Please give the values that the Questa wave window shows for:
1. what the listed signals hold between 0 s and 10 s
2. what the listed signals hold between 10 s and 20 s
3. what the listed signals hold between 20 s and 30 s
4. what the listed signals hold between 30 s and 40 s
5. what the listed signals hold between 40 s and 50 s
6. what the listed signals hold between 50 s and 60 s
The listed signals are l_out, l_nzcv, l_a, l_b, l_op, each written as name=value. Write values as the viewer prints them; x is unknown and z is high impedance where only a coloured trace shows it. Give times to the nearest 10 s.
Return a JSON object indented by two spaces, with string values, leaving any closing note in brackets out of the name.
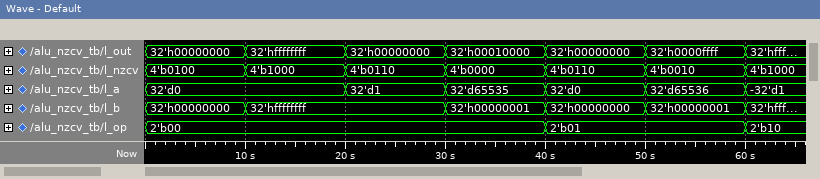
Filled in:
{
  "what the listed signals hold between 0 s and 10 s": "l_out=32'h00000000, l_nzcv=4'b0100, l_a=32'd0, l_b=32'h00000000, l_op=2'b00",
  "what the listed signals hold between 10 s and 20 s": "l_out=32'hffffffff, l_nzcv=4'b1000, l_a=32'd0, l_b=32'hffffffff, l_op=2'b00",
  "what the listed signals hold between 20 s and 30 s": "l_out=32'h00000000, l_nzcv=4'b0110, l_a=32'd1, l_b=32'hffffffff, l_op=2'b00",
  "what the listed signals hold between 30 s and 40 s": "l_out=32'h00010000, l_nzcv=4'b0000, l_a=32'd65535, l_b=32'h00000001, l_op=2'b00",
  "what the listed signals hold between 40 s and 50 s": "l_out=32'h00000000, l_nzcv=4'b0110, l_a=32'd0, l_b=32'h00000000, l_op=2'b01",
  "what the listed signals hold between 50 s and 60 s": "l_out=32'h0000ffff, l_nzcv=4'b0010, l_a=32'd65536, l_b=32'h00000001, l_op=2'b01"
}
